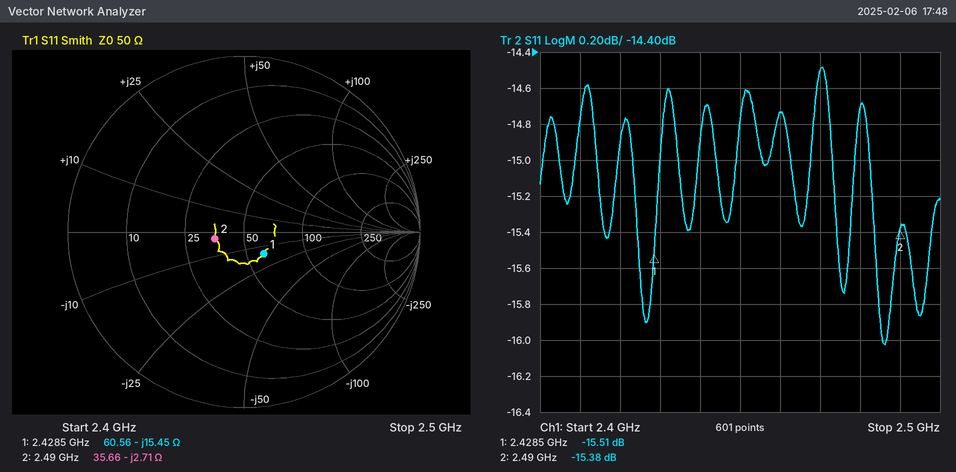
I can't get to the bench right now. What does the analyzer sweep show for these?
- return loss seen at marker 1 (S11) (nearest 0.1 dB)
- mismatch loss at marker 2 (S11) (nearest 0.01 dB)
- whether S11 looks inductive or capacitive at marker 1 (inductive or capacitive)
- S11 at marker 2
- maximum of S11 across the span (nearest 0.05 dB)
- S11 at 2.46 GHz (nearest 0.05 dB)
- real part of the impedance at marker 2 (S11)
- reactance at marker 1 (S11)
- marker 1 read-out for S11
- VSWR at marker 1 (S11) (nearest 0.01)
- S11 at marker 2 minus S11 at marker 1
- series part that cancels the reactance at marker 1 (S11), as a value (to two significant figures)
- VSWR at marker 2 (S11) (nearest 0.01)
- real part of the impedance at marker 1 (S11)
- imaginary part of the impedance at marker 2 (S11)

15.5 dB
0.13 dB
capacitive
-15.38 dB
-14.50 dB
-14.75 dB
35.66 Ω
-15.45 Ω
-15.51 dB
1.40
0.13 dB
1.0 nH
1.41
60.56 Ω
-2.71 Ω
